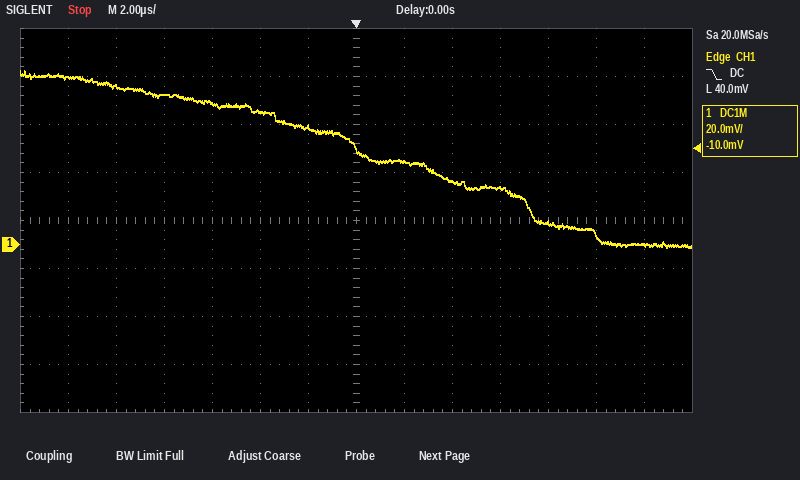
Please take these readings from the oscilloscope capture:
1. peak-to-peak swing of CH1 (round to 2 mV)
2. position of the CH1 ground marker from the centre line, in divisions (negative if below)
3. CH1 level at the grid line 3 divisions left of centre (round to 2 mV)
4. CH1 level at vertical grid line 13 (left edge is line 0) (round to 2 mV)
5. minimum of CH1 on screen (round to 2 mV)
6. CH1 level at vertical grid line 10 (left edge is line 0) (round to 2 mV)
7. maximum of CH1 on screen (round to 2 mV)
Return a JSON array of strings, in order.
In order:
["74 mV", "-0.5 div", "58 mV", "0 mV", "-2 mV", "24 mV", "72 mV"]
